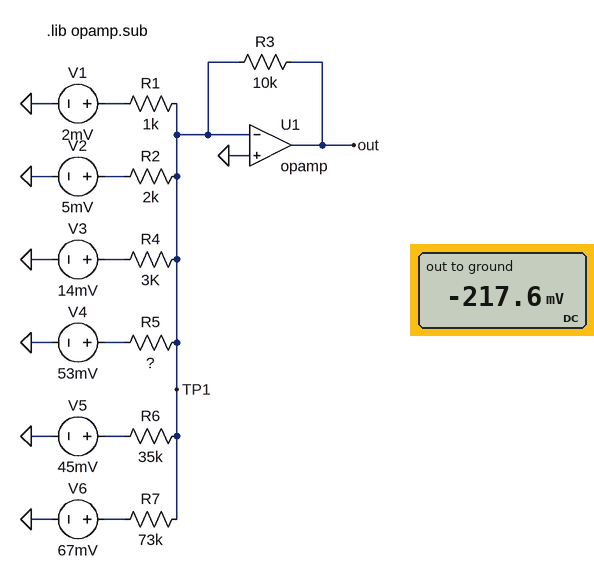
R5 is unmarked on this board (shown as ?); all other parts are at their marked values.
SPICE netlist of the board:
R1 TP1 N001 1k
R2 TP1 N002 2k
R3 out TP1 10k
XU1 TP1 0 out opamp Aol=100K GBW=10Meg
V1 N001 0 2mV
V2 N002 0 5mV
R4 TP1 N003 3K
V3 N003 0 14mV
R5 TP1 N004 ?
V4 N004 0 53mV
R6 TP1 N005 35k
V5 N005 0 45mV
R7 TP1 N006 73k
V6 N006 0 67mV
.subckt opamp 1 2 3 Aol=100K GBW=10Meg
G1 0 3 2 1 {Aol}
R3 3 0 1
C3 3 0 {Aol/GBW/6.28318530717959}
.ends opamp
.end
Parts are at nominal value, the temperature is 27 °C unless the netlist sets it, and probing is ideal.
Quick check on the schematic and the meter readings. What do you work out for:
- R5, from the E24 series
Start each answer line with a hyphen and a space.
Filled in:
- 5.1 kΩ
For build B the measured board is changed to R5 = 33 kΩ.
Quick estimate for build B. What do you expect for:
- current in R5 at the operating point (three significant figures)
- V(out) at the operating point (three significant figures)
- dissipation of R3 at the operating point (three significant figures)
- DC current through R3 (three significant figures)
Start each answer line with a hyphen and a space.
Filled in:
- 1.61 µA
- -130 mV
- 1.68 µW
- 13.0 µA
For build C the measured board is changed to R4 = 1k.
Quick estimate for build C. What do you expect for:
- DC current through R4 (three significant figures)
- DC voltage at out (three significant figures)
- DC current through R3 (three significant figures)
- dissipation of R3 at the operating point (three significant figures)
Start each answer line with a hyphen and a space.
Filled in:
- 14.0 µA
- -311 mV
- 31.1 µA
- 9.66 µW
